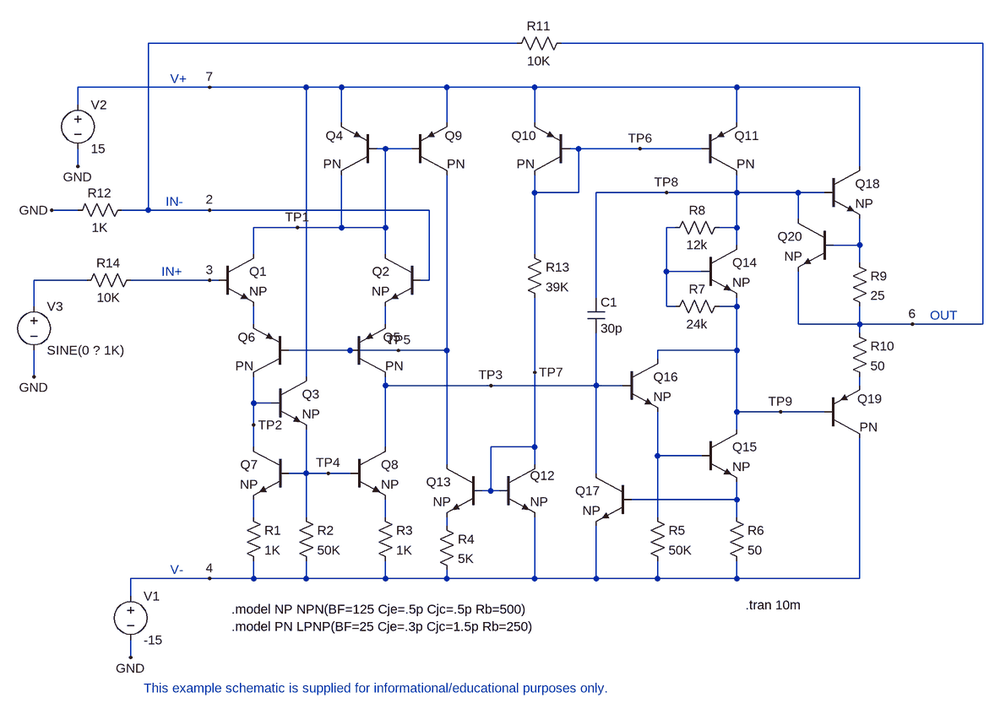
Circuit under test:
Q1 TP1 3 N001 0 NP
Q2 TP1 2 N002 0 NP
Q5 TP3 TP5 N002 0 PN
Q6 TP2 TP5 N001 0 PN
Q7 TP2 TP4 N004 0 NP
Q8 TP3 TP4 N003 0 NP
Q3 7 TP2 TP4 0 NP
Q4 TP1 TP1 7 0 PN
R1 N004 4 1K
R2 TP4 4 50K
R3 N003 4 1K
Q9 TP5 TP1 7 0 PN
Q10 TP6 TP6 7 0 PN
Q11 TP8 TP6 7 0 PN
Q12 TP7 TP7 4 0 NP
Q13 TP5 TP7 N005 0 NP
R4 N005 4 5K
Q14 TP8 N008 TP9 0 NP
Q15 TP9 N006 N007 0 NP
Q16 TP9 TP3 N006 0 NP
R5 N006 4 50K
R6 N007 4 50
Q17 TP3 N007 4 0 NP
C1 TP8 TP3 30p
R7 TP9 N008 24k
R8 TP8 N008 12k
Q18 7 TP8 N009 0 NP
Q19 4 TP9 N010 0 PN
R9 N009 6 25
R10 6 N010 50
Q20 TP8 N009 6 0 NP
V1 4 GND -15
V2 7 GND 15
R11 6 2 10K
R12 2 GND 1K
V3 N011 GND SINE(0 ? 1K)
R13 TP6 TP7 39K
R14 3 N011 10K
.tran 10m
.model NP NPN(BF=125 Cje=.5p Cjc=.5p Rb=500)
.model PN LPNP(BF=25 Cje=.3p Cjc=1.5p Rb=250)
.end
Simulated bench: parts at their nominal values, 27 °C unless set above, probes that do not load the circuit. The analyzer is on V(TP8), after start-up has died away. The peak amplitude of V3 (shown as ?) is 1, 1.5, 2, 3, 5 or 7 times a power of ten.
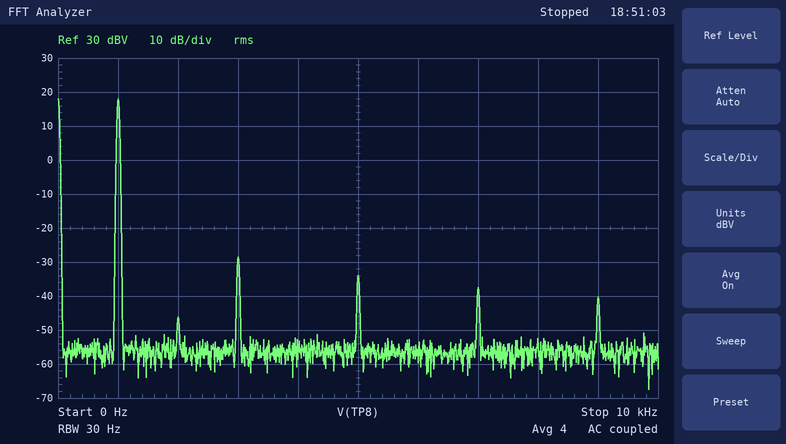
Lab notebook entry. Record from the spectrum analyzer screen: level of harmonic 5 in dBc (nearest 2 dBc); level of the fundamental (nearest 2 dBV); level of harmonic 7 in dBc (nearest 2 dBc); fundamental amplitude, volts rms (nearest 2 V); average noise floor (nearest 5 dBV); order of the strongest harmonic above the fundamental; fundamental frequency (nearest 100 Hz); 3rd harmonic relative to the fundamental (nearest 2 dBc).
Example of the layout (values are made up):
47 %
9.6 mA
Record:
-52 dBc
18 dBV
-56 dBc
8 V
-55 dBV
3
1.0 kHz
-46 dBc
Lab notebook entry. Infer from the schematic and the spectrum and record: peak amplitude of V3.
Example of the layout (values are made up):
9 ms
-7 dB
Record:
1 V
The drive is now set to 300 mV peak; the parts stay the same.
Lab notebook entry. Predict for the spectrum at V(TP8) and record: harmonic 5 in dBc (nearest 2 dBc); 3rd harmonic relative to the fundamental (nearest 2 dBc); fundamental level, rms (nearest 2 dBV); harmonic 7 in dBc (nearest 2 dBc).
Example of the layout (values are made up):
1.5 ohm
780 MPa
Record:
-44 dBc
-38 dBc
8 dBV
-48 dBc
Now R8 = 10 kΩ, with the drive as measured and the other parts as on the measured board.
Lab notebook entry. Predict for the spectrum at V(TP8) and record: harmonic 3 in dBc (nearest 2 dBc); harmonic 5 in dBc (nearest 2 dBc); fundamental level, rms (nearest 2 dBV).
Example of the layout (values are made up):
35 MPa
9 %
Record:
-44 dBc
-50 dBc
18 dBV
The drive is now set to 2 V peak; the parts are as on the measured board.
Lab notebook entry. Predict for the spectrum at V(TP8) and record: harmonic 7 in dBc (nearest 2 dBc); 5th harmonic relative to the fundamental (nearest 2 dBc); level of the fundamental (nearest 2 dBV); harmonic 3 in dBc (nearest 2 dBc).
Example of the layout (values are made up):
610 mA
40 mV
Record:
-32 dBc
-54 dBc
22 dBV
-16 dBc
